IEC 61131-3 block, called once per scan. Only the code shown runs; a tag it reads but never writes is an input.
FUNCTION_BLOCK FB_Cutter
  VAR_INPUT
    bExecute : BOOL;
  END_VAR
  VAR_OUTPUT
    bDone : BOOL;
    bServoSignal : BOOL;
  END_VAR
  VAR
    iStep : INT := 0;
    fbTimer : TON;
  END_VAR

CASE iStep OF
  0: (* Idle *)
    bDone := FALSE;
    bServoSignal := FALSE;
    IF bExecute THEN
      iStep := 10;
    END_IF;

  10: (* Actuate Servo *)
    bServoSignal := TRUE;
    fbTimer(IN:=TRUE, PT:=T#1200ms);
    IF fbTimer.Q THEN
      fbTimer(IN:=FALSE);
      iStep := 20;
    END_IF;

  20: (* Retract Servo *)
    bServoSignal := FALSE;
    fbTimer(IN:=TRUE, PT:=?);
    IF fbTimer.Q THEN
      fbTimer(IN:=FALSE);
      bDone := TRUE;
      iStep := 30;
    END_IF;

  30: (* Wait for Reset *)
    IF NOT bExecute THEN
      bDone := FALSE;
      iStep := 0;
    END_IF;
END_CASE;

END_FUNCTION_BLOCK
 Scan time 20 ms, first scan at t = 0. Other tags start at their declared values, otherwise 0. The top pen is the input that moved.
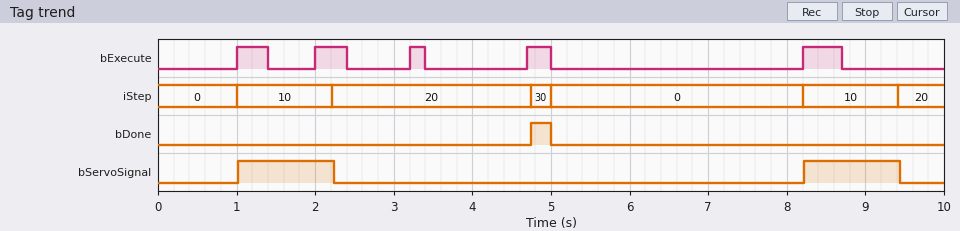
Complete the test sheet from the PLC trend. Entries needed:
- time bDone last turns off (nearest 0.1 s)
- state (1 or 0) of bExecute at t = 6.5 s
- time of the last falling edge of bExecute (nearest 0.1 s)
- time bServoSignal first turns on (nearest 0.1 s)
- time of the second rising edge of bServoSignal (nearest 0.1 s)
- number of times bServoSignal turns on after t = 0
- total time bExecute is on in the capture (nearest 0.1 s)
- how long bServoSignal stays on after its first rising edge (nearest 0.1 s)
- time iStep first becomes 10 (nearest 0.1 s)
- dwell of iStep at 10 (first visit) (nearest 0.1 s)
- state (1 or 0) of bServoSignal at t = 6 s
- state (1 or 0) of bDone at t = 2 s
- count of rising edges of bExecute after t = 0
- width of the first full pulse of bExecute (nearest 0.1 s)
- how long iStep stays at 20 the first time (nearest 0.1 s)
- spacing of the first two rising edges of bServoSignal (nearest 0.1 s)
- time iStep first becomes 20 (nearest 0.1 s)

5.0 s
0
8.7 s
1.0 s
8.2 s
2
1.8 s
1.2 s
1.0 s
1.2 s
0
0
5
0.4 s
2.5 s
7.2 s
2.2 s
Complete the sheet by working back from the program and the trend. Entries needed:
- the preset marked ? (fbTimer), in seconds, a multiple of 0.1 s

2.5 s
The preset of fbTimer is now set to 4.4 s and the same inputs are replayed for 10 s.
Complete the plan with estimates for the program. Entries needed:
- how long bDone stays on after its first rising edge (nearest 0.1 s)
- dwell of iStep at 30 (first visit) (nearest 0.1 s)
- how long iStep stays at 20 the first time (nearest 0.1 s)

0.0 s
0.0 s
4.4 s
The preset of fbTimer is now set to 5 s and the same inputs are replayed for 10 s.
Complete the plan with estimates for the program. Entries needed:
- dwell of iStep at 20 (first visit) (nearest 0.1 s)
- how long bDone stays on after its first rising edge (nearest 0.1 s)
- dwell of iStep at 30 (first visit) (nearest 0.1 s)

5.0 s
0.0 s
0.0 s
